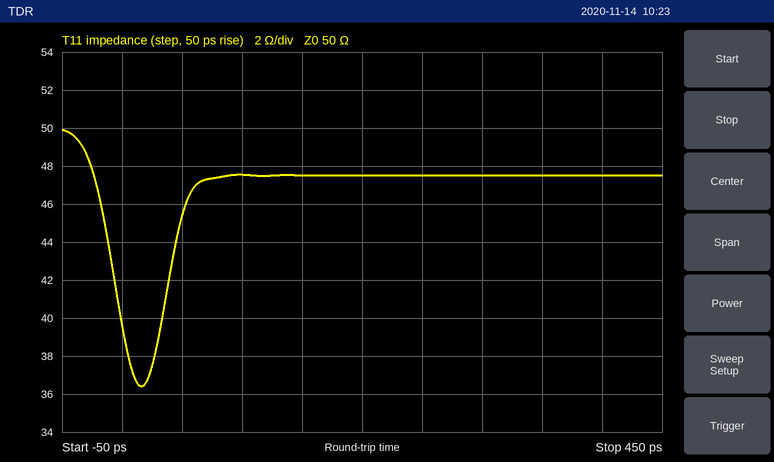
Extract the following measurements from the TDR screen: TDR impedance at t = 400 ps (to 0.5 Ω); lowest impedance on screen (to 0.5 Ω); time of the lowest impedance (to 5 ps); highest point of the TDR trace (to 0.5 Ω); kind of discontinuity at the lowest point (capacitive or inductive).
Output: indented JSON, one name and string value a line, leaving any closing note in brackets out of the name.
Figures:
{
  "TDR impedance at t = 400 ps": "47.5 Ω",
  "lowest impedance on screen": "36.5 Ω",
  "time of the lowest impedance": "15 ps",
  "highest point of the TDR trace": "50.0 Ω",
  "kind of discontinuity at the lowest point": "capacitive"
}
